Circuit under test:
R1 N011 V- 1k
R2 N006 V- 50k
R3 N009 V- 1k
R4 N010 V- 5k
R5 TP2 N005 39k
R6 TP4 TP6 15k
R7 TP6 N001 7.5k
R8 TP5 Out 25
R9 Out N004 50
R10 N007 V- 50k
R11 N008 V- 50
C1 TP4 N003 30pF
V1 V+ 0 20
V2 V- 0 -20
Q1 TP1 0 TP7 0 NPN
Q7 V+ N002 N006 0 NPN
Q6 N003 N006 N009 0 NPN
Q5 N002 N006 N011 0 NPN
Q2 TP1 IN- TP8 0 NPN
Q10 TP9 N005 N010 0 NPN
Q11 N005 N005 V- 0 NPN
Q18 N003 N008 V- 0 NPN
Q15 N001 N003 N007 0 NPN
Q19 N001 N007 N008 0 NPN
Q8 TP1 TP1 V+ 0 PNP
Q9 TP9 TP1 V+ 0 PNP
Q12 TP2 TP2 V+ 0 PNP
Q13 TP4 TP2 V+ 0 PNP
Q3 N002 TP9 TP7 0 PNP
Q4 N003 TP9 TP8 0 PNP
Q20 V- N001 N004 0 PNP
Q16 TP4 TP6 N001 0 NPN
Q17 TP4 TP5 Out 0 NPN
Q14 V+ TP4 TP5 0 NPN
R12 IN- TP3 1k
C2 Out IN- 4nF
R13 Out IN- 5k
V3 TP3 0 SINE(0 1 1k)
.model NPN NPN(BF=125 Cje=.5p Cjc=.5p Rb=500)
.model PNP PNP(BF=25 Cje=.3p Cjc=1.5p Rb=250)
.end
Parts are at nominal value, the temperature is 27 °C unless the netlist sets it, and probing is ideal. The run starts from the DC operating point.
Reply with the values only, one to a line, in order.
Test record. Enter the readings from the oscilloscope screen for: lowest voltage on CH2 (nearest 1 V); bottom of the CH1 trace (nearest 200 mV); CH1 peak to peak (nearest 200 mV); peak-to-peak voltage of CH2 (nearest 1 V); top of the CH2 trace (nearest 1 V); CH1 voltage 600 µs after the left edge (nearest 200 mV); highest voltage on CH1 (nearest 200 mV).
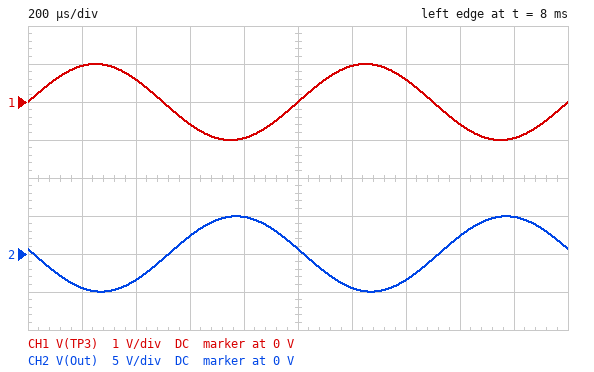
-5 V
-1.0 V
2.0 V
10 V
5 V
-600 mV
1.0 V
